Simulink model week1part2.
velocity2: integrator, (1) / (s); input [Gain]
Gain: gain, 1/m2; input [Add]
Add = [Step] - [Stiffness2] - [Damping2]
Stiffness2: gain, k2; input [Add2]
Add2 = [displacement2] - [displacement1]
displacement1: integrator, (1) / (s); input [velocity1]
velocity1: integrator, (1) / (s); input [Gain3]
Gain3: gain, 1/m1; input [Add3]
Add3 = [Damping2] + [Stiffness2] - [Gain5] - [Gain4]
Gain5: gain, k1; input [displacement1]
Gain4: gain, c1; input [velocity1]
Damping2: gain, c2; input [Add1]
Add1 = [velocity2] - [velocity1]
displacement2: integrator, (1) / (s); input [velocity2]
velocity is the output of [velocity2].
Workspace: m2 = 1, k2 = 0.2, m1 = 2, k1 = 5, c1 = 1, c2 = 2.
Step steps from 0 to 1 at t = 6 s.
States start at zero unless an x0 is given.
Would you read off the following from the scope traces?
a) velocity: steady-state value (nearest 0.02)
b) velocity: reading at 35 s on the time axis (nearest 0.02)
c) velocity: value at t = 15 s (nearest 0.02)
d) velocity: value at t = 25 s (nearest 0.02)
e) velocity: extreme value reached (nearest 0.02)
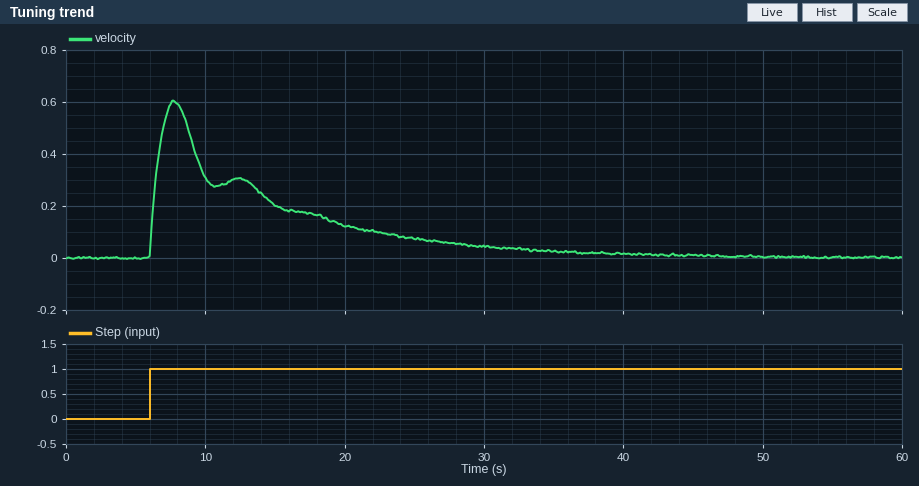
0.00
0.02
0.20
0.08
0.60
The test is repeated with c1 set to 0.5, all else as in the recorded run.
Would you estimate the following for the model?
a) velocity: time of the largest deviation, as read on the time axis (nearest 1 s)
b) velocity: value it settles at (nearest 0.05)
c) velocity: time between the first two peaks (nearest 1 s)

8 s
0.00
5 s
